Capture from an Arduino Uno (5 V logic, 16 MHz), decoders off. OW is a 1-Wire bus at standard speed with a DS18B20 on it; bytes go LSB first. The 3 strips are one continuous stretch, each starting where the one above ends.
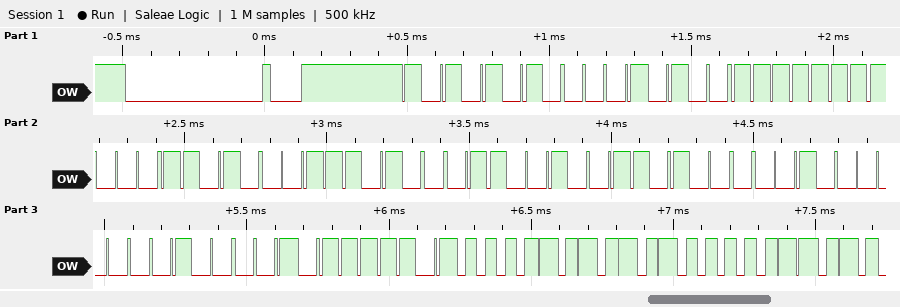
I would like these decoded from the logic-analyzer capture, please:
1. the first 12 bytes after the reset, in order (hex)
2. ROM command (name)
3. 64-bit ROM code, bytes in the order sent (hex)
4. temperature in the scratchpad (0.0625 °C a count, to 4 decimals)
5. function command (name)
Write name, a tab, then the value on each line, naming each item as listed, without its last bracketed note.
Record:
the first 12 bytes after the reset, in order	55 28 FF 58 5C 4C 16 04 84 BE 50 05
ROM command	Match ROM
64-bit ROM code, bytes in the order sent	28 FF 58 5C 4C 16 04 84
temperature in the scratchpad	85.0000 °C
function command	Read Scratchpad
